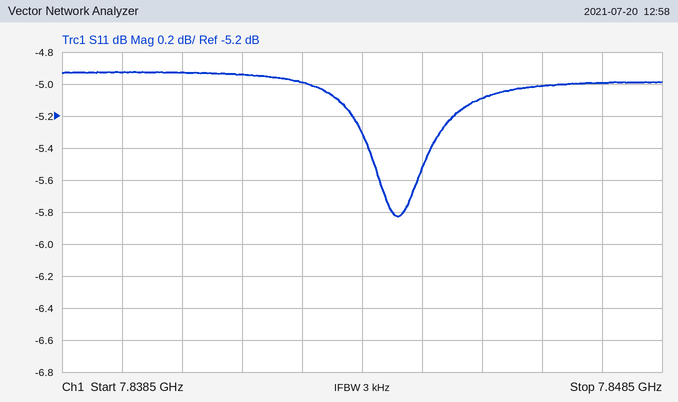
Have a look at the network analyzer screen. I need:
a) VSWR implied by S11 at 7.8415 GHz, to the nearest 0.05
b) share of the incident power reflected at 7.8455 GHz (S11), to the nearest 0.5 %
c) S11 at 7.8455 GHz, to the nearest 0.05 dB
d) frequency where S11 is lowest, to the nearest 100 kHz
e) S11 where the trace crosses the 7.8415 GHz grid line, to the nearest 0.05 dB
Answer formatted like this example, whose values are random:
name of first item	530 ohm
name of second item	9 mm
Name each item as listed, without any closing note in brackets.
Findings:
VSWR implied by S11 at 7.8415 GHz, to the nearest 0.05	3.60
share of the incident power reflected at 7.8455 GHz (S11), to the nearest 0.5 %	31.0 %
S11 at 7.8455 GHz, to the nearest 0.05 dB	-5.10 dB
frequency where S11 is lowest, to the nearest 100 kHz	7.8441 GHz
S11 where the trace crosses the 7.8415 GHz grid line, to the nearest 0.05 dB	-4.95 dB
